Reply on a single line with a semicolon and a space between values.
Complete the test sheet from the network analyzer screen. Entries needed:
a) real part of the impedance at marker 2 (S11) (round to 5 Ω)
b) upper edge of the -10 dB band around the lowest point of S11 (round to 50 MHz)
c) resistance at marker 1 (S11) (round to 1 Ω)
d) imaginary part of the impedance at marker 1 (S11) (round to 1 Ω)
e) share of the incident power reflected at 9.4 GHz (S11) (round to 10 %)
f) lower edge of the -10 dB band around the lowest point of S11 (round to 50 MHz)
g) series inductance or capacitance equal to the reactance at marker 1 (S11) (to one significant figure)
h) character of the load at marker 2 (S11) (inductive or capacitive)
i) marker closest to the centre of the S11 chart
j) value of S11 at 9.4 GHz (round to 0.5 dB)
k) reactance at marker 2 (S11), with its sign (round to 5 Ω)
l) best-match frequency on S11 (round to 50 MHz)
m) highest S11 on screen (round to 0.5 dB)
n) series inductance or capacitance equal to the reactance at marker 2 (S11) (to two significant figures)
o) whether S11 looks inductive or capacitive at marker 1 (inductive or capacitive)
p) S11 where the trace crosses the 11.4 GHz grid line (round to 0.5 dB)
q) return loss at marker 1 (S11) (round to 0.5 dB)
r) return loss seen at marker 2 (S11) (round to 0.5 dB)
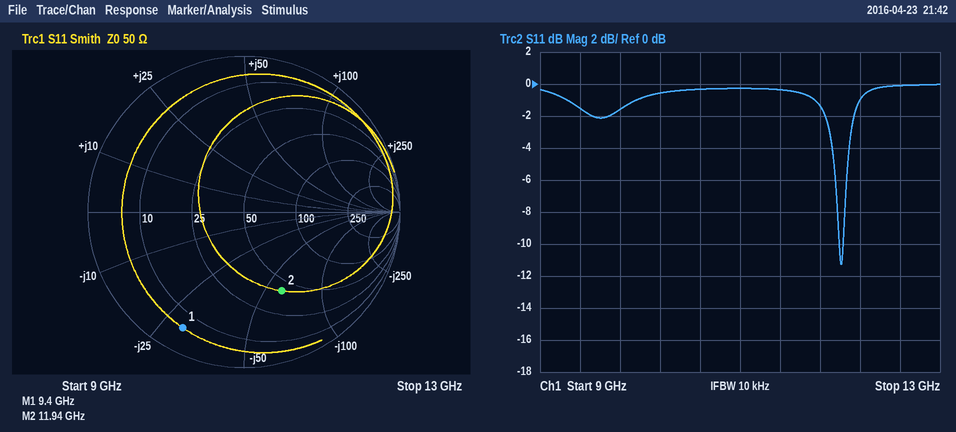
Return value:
40 Ω; 12.05 GHz; 6 Ω; -30 Ω; 70 %; 12.00 GHz; 600 fF; capacitive; marker 2; -1.5 dB; -60 Ω; 12.00 GHz; 0.0 dB; 220 fF; capacitive; -0.5 dB; 1.5 dB; 5.0 dB
